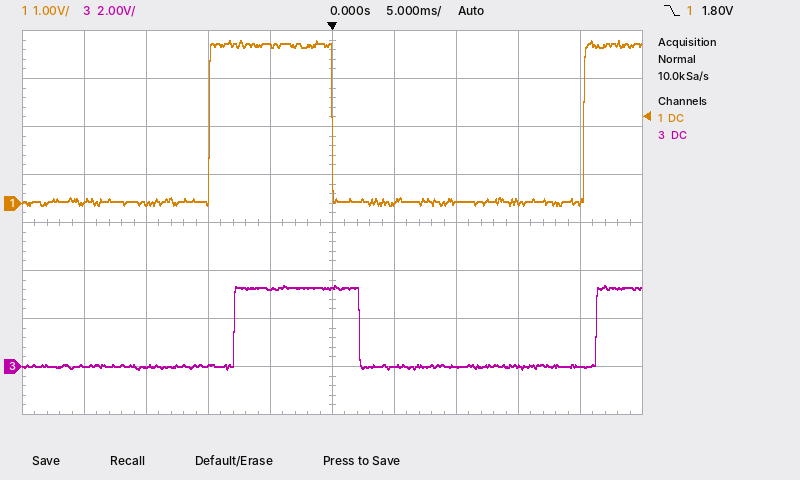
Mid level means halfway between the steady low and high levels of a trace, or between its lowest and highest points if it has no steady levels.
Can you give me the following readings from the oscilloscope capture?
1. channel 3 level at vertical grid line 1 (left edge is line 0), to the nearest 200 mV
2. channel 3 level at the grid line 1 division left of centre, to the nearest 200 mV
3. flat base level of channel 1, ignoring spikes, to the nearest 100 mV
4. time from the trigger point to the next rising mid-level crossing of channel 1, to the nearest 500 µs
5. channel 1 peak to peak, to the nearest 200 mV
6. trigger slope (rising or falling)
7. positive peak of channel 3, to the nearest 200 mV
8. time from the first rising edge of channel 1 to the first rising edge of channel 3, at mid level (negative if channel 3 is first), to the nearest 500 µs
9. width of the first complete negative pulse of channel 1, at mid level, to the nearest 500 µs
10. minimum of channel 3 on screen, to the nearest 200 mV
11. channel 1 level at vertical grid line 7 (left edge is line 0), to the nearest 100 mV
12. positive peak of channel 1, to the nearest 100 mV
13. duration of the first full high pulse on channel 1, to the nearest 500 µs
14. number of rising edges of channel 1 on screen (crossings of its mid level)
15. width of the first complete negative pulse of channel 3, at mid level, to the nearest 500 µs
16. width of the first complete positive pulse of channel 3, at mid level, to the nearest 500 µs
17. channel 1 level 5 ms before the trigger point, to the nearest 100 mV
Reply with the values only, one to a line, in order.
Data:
0.0 V
3.2 V
0.0 V
20.5 ms
3.4 V
falling
3.4 V
+2.0 ms
20.5 ms
-200 mV
0.0 V
3.4 V
10.0 ms
2
19.0 ms
10.0 ms
3.3 V
